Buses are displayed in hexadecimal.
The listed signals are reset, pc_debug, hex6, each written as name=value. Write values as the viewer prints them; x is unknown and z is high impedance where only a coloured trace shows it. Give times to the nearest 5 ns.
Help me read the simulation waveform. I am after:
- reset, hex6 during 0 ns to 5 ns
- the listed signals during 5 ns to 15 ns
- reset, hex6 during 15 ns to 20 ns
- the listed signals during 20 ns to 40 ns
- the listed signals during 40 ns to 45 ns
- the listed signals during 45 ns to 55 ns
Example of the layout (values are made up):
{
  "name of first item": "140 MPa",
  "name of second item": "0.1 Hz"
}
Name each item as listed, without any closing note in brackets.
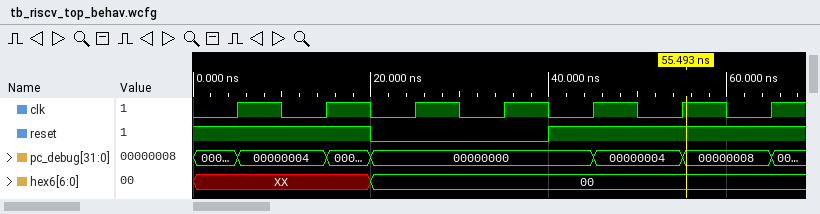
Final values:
{
  "reset, hex6 during 0 ns to 5 ns": "reset=1, hex6=XX",
  "the listed signals during 5 ns to 15 ns": "reset=1, pc_debug=00000004, hex6=XX",
  "reset, hex6 during 15 ns to 20 ns": "reset=1, hex6=XX",
  "the listed signals during 20 ns to 40 ns": "reset=0, pc_debug=00000000, hex6=00",
  "the listed signals during 40 ns to 45 ns": "reset=1, pc_debug=00000000, hex6=00",
  "the listed signals during 45 ns to 55 ns": "reset=1, pc_debug=00000004, hex6=00"
}
